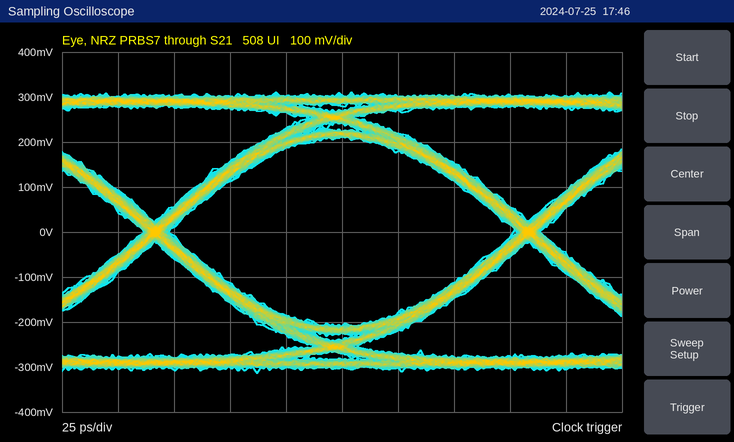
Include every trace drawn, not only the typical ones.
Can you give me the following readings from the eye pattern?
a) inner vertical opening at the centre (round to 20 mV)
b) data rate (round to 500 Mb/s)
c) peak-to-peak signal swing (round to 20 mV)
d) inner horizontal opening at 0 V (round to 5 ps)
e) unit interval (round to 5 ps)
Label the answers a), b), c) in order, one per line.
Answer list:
a) 420 mV
b) 6.0 Gb/s
c) 620 mV
d) 155 ps
e) 165 ps
